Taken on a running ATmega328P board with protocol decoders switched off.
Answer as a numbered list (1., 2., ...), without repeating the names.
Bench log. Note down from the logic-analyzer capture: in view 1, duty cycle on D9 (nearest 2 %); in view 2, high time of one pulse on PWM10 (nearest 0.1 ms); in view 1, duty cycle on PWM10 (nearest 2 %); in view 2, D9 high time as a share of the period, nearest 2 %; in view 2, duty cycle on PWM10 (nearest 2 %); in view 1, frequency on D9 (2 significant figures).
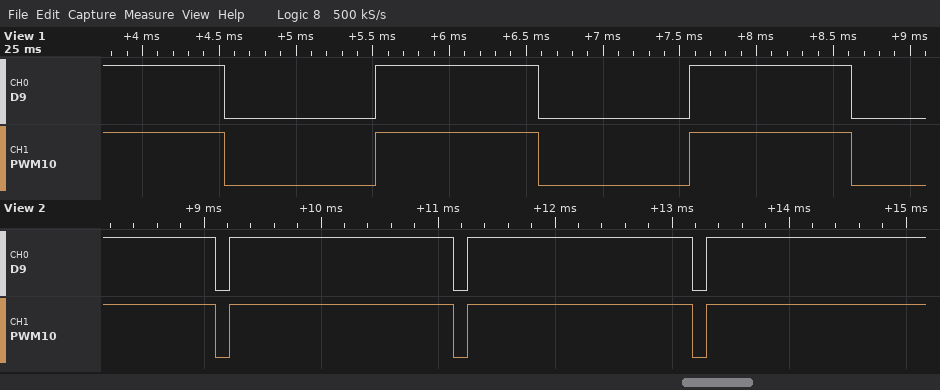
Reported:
1. 52 %
2. 1.9 ms
3. 52 %
4. 94 %
5. 94 %
6. 490 Hz
